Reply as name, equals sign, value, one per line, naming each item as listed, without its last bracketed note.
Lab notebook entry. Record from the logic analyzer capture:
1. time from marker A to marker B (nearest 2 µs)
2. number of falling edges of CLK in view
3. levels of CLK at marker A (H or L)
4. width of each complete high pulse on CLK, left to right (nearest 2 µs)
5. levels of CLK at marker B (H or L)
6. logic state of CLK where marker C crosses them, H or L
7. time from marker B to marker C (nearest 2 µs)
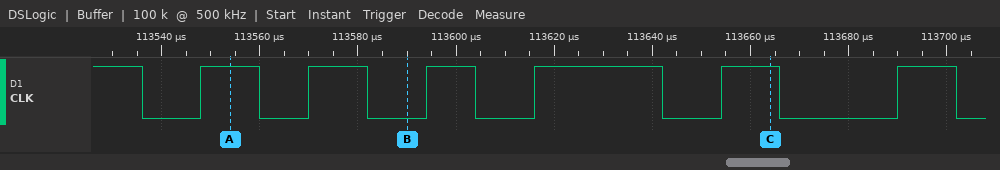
time from marker A to marker B = 36 µs
number of falling edges of CLK in view = 7
levels of CLK at marker A = CLK=H
width of each complete high pulse on CLK, left to right = 12 µs, 12 µs, 10 µs, 26 µs, 12 µs, 12 µs
levels of CLK at marker B = CLK=L
logic state of CLK where marker C crosses them, H or L = CLK=H
time from marker B to marker C = 74 µs
